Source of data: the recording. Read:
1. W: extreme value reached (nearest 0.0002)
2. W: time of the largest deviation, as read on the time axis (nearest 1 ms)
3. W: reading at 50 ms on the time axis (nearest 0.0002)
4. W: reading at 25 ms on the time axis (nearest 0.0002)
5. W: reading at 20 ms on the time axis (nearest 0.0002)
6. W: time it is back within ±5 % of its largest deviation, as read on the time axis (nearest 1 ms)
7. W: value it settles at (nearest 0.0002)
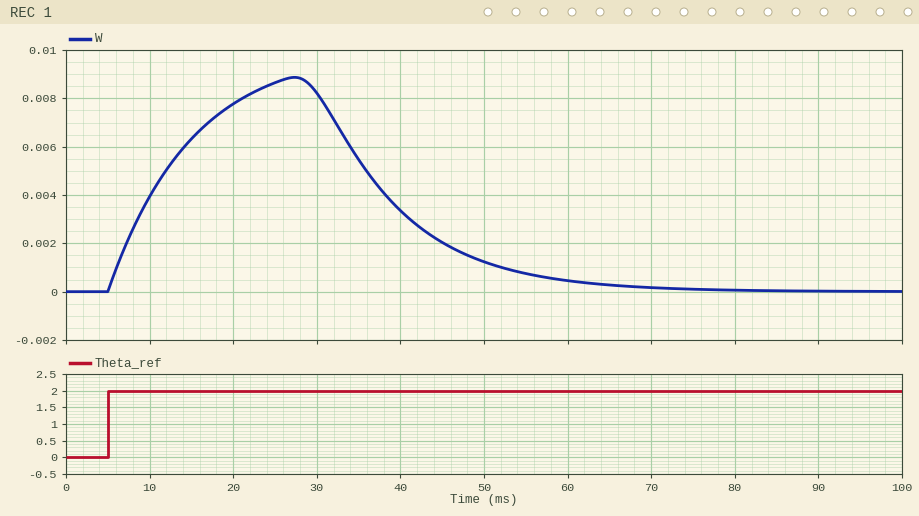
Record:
0.0088
27 ms
0.0012
0.0086
0.0078
60 ms
0.0000
